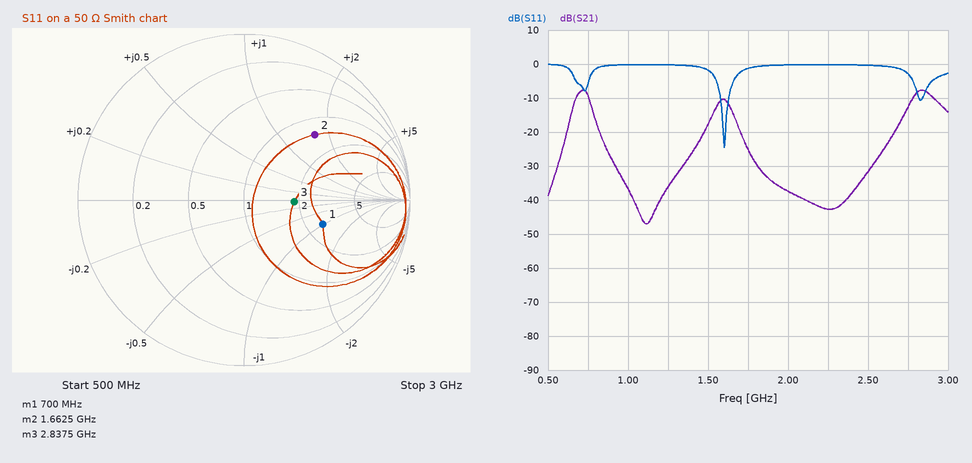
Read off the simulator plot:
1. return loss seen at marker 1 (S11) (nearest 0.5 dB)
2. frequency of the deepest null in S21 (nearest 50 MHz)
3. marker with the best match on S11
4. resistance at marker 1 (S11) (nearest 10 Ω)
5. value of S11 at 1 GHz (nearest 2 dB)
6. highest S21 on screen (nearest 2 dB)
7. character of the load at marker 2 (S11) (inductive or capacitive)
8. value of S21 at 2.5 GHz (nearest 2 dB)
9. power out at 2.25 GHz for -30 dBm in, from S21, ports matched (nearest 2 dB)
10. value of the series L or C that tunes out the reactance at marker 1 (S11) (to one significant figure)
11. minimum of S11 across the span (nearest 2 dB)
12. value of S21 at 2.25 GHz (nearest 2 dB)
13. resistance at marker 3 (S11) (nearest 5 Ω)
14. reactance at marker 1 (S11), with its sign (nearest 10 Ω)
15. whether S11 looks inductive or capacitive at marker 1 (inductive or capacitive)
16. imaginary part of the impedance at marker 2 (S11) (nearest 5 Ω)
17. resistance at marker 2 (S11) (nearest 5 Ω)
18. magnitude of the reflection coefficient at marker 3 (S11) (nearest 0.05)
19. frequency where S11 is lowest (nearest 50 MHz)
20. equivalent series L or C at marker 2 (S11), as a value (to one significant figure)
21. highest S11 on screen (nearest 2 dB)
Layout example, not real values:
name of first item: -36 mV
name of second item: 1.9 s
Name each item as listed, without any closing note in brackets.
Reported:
return loss seen at marker 1 (S11): 6.0 dB
frequency of the deepest null in S21: 1.10 GHz
marker with the best match on S11: marker 3
resistance at marker 1 (S11): 130 Ω
value of S11 at 1 GHz: 0 dB
highest S21 on screen: -8 dB
character of the load at marker 2 (S11): inductive
value of S21 at 2.5 GHz: -32 dB
power out at 2.25 GHz for -30 dBm in, from S21, ports matched: -72 dBm
value of the series L or C that tunes out the reactance at marker 1 (S11): 10 nH
minimum of S11 across the span: -24 dB
value of S21 at 2.25 GHz: -42 dB
resistance at marker 3 (S11): 95 Ω
reactance at marker 1 (S11), with its sign: -50 Ω
whether S11 looks inductive or capacitive at marker 1: capacitive
imaginary part of the impedance at marker 2 (S11): +80 Ω
resistance at marker 2 (S11): 70 Ω
magnitude of the reflection coefficient at marker 3 (S11): 0.30
frequency where S11 is lowest: 1.60 GHz
equivalent series L or C at marker 2 (S11), as a value: 8 nH
highest S11 on screen: 0 dB
